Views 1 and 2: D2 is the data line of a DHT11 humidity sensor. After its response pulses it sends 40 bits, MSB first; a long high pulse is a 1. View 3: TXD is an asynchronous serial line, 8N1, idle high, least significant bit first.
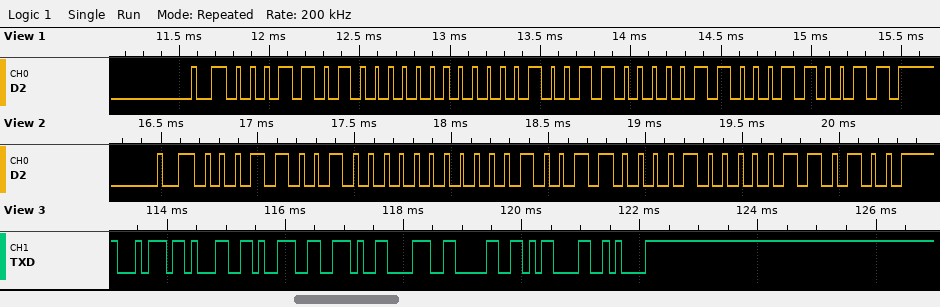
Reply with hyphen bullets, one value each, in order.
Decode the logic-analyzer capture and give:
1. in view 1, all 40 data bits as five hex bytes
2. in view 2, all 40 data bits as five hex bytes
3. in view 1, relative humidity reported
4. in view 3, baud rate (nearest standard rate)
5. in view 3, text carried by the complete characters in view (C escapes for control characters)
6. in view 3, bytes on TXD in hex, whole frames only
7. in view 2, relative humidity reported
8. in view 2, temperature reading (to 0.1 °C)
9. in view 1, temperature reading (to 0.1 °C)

- 1A 00 13 06 33
- 19 00 13 08 34
- 26 %
- 9600 baud
- "t19.80\r\n"
- 74 31 39 2E 38 30 0D 0A
- 25 %
- 19.8 °C
- 19.6 °C
